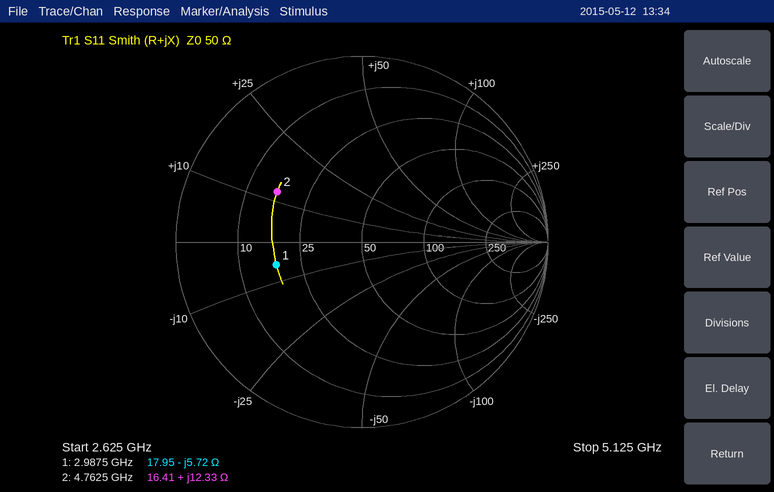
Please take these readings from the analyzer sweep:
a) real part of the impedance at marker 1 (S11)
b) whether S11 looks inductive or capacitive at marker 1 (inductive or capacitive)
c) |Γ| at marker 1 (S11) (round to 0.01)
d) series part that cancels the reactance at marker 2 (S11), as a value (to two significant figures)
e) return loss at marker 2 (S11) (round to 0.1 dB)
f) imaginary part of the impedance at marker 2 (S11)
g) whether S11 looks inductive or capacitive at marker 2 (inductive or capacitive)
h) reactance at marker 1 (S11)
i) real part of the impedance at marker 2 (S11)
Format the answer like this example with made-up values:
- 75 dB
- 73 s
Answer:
- 17.95 Ω
- capacitive
- 0.48
- 2.7 pF
- 5.5 dB
- +12.33 Ω
- inductive
- -5.72 Ω
- 16.41 Ω
